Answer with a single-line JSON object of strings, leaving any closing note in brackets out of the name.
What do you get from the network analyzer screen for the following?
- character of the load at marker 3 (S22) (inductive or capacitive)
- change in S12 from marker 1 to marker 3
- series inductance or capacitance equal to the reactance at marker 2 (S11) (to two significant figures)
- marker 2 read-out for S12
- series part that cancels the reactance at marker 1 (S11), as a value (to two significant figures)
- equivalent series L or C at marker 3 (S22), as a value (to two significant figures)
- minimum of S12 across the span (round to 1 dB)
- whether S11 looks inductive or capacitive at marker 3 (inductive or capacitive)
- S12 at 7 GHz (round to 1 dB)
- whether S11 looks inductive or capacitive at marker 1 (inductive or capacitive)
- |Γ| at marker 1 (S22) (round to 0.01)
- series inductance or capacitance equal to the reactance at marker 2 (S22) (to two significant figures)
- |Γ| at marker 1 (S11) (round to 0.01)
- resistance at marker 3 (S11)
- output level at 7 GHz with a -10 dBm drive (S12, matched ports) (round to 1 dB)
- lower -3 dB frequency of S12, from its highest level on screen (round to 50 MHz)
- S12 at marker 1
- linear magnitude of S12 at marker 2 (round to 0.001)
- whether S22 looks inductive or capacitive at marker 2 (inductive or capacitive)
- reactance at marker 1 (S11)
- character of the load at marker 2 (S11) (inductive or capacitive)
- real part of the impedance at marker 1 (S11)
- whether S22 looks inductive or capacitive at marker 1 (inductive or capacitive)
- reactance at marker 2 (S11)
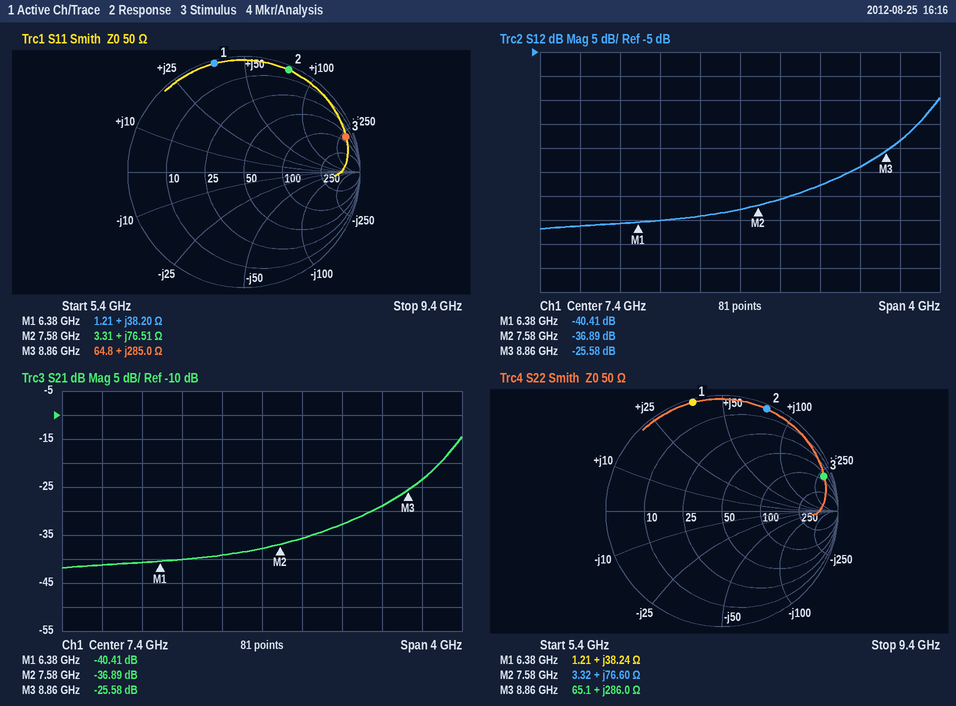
{"character of the load at marker 3 (S22)": "inductive", "change in S12 from marker 1 to marker 3": "14.83 dB", "series inductance or capacitance equal to the reactance at marker 2 (S11)": "1.6 nH", "marker 2 read-out for S12": "-36.89 dB", "series part that cancels the reactance at marker 1 (S11), as a value": "650 fF", "equivalent series L or C at marker 3 (S22), as a value": "5.1 nH", "minimum of S12 across the span": "-42 dB", "whether S11 looks inductive or capacitive at marker 3": "inductive", "S12 at 7 GHz": "-39 dB", "whether S11 looks inductive or capacitive at marker 1": "inductive", "|Γ| at marker 1 (S22)": "0.97", "series inductance or capacitance equal to the reactance at marker 2 (S22)": "1.6 nH", "|Γ| at marker 1 (S11)": "0.97", "resistance at marker 3": "64.8 Ω", "output level at 7 GHz with a -10 dBm drive (S12, matched ports)": "-49 dBm", "lower -3 dB frequency of S12, from its highest level on screen": "9.30 GHz", "S12 at marker 1": "-40.41 dB", "linear magnitude of S12 at marker 2": "0.014", "whether S22 looks inductive or capacitive at marker 2": "inductive", "reactance at marker 1": "+38.20 Ω", "character of the load at marker 2 (S11)": "inductive", "real part of the impedance at marker 1": "1.21 Ω", "whether S22 looks inductive or capacitive at marker 1": "inductive", "reactance at marker 2": "+76.51 Ω"}
